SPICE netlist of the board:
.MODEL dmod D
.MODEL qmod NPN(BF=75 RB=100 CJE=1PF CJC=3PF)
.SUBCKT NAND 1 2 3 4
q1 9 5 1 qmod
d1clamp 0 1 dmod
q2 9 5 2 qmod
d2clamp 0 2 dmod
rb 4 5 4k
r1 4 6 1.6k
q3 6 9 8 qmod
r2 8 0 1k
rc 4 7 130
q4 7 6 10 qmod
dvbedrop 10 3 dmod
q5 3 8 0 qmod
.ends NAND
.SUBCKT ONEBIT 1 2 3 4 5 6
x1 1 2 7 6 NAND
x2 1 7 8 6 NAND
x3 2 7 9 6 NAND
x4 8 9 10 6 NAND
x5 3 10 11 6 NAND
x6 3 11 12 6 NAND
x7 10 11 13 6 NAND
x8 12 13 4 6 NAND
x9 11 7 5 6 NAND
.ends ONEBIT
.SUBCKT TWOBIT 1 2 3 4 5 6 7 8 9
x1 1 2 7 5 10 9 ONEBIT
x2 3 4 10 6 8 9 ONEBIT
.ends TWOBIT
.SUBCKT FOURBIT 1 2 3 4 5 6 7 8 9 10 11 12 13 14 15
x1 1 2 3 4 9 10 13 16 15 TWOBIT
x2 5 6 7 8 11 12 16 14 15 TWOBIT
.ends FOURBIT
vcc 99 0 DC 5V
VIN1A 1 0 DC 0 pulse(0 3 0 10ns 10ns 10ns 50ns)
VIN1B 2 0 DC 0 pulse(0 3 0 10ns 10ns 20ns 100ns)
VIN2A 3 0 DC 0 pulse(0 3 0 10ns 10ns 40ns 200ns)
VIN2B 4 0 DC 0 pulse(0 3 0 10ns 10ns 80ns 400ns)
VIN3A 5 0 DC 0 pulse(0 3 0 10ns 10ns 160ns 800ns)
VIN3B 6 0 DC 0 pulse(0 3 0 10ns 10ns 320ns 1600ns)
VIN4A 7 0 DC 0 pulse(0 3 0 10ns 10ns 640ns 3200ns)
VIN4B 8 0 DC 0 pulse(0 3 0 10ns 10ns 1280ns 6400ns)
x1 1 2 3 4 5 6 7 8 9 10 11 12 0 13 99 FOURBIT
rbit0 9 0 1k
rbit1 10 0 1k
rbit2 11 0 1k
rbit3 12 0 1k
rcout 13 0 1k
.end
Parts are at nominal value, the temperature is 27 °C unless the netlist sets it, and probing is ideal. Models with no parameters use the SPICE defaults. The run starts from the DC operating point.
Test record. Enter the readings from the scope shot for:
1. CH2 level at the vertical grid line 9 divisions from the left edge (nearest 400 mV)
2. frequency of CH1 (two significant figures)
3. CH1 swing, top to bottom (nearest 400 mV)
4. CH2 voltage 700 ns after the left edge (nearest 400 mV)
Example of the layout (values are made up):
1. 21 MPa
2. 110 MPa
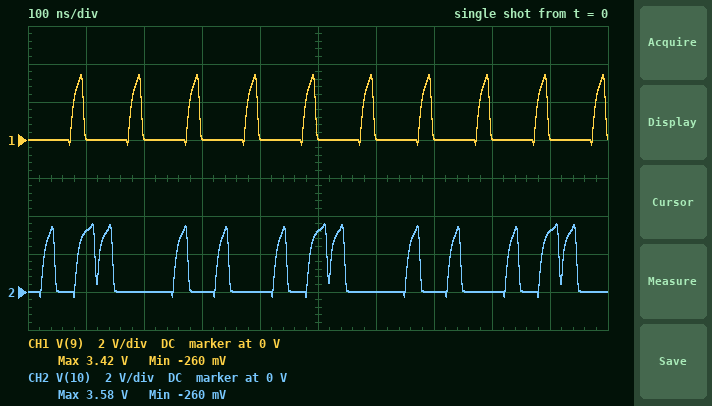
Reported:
1. 3.2 V
2. 10 MHz
3. 3.6 V
4. 0 V
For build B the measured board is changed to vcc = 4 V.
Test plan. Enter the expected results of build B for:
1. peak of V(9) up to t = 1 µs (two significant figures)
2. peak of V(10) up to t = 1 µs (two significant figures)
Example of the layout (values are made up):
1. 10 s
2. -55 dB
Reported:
1. 2.5 V
2. 2.6 V
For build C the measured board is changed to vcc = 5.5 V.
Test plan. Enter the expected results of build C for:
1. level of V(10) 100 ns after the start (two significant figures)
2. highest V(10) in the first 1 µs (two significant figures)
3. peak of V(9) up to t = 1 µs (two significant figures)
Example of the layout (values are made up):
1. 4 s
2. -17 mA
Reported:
1. 3.7 V
2. 4.1 V
3. 3.9 V
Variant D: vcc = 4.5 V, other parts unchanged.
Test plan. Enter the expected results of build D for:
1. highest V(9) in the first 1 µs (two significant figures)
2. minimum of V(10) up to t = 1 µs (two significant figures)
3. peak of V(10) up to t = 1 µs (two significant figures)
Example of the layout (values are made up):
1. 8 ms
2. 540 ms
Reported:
1. 3.0 V
2. -270 mV
3. 3.1 V
